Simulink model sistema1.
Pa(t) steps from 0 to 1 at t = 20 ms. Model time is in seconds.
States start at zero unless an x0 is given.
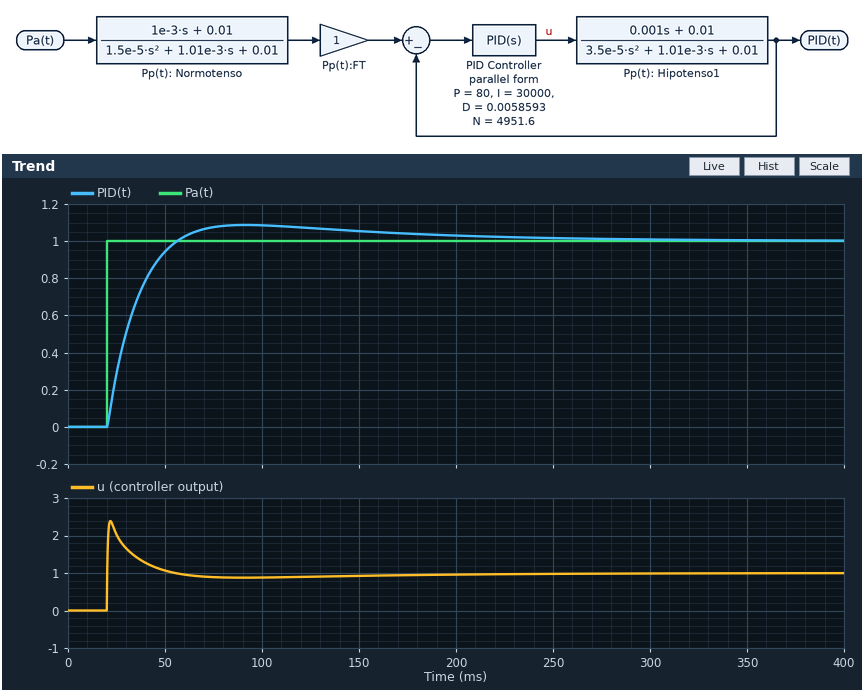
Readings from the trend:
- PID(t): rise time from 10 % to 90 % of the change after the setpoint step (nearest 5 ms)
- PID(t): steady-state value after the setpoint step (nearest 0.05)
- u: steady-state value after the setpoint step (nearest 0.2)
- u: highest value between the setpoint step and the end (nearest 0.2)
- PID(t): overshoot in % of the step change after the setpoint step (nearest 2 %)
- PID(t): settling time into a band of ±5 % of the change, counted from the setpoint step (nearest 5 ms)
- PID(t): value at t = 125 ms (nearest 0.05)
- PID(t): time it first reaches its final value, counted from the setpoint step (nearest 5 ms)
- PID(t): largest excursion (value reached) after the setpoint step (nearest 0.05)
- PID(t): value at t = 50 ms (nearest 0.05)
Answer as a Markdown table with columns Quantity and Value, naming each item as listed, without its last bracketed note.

| Quantity | Value |
|---|---|
| PID(t): rise time from 10 % to 90 % of the change after the setpoint step | 25 ms |
| PID(t): steady-state value after the setpoint step | 1.00 |
| u: steady-state value after the setpoint step | 1.0 |
| u: highest value between the setpoint step and the end | 2.4 |
| PID(t): overshoot in % of the step change after the setpoint step | 8 % |
| PID(t): settling time into a band of ±5 % of the change, counted from the setpoint step | 135 ms |
| PID(t): value at t = 125 ms | 1.05 |
| PID(t): time it first reaches its final value, counted from the setpoint step | 35 ms |
| PID(t): largest excursion (value reached) after the setpoint step | 1.10 |
| PID(t): value at t = 50 ms | 0.95 |
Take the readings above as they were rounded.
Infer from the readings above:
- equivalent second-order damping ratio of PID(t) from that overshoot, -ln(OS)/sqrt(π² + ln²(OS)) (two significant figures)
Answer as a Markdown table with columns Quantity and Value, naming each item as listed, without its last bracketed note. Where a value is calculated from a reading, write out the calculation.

| Quantity | Value |
|---|---|
| equivalent second-order damping ratio of PID(t) from that overshoot, -ln(OS)/sqrt(π² + ln²(OS)) | ln(0.08) = -2.526; 2.526 / sqrt(9.870 + 6.379) = 0.63 |
